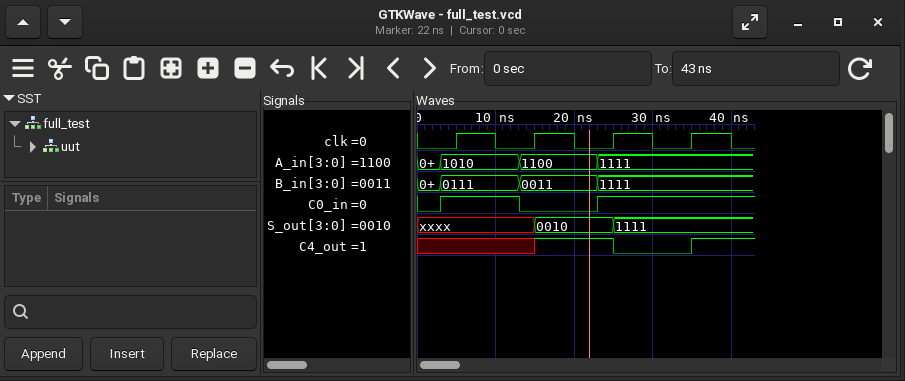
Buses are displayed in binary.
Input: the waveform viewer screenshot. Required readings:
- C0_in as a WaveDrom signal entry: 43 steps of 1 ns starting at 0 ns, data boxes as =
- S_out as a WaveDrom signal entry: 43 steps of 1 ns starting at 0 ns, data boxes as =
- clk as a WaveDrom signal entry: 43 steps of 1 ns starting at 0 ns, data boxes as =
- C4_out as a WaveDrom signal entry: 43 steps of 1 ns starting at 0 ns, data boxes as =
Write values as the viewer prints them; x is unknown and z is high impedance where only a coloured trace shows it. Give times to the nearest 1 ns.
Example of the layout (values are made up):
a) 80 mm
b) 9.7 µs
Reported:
a) {name: 'C0_in', wave: '0..1.........0.........1...................'}
b) {name: 'S_out', wave: 'x..............=.........=.................', data: '0010 1111'}
c) {name: 'clk', wave: '0....1....0....1....0....1....0....1....0..'}
d) {name: 'C4_out', wave: 'x..............1.........0.........1.......'}
